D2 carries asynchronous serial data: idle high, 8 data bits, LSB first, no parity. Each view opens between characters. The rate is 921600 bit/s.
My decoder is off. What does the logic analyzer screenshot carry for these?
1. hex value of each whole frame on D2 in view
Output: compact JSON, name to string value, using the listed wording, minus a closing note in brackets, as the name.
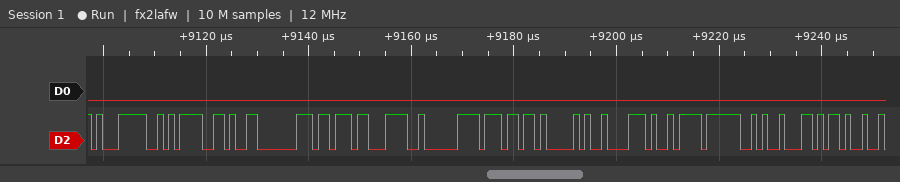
{"hex value of each whole frame on D2 in view": "F1, EA, 96, C0, BB, 3C, E0, B7, 41, C2, E9, 3F, 89, 2D"}
